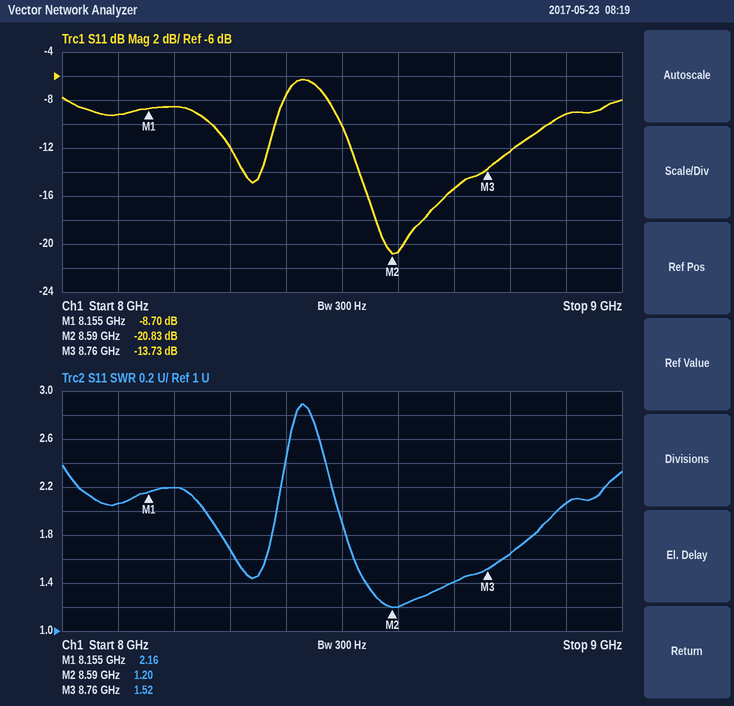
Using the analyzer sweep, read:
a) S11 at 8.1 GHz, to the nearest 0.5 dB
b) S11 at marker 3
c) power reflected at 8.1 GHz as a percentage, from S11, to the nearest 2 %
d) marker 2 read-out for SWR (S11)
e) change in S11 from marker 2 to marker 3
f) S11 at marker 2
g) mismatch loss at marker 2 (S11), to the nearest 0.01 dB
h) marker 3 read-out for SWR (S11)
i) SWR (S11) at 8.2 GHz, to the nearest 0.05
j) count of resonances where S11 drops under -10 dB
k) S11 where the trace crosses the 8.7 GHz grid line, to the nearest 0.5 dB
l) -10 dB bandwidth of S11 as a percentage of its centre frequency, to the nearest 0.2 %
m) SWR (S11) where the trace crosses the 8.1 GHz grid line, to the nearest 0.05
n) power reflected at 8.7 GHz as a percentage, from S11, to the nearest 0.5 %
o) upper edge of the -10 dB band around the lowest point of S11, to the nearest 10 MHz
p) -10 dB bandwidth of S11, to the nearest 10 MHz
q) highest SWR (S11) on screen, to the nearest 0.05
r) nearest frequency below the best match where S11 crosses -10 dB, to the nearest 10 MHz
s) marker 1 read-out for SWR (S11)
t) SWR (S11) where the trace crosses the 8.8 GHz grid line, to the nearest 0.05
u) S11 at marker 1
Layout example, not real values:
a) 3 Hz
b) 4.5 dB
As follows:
a) -9.0 dB
b) -13.73 dB
c) 12 %
d) 1.20
e) 7.10 dB
f) -20.83 dB
g) 0.04 dB
h) 1.52
i) 2.20
j) 2
k) -15.5 dB
l) 4.2 %
m) 2.05
n) 3.0 %
o) 8.87 GHz
p) 370 MHz
q) 2.90
r) 8.50 GHz
s) 2.16
t) 1.65
u) -8.70 dB
